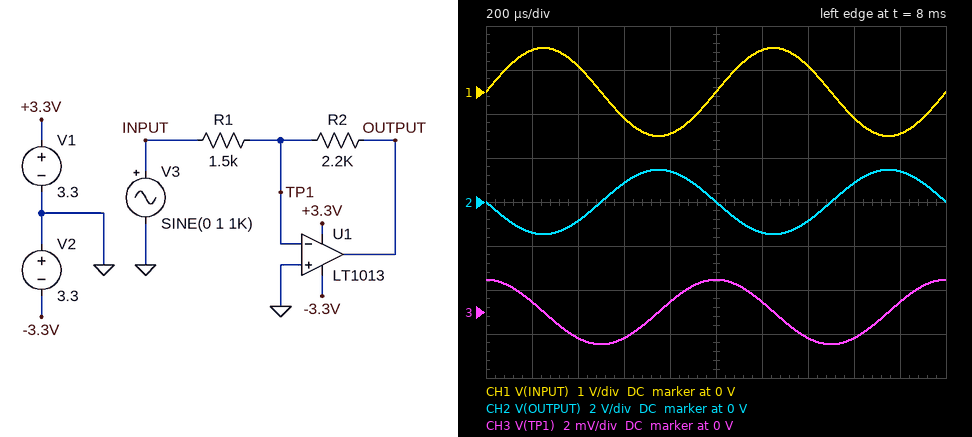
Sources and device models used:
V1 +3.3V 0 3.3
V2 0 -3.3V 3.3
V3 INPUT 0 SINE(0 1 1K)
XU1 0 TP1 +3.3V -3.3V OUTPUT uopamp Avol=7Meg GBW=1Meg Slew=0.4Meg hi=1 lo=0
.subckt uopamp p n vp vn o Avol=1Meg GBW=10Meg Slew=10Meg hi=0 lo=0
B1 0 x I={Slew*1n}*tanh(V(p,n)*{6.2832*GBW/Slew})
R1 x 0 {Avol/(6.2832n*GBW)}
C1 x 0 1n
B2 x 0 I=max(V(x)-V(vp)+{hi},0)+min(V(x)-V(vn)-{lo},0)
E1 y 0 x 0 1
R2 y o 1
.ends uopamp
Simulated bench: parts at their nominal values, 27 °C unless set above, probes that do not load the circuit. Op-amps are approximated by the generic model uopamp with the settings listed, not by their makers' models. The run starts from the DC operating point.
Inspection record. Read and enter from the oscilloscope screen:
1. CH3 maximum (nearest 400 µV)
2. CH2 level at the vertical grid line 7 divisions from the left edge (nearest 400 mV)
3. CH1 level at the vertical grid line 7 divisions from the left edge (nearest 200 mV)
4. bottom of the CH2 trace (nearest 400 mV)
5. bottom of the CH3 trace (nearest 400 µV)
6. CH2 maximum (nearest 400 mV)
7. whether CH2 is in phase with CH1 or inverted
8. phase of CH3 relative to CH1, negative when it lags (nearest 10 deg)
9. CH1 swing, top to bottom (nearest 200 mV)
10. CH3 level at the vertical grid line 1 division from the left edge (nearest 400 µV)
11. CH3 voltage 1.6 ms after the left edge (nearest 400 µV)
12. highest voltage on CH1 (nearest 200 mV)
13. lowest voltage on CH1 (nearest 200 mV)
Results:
1.6 mV
-800 mV
600 mV
-1.6 V
-1.6 mV
1.6 V
inverted
90 deg
2.0 V
400 µV
-1.2 mV
1.0 V
-1.0 V
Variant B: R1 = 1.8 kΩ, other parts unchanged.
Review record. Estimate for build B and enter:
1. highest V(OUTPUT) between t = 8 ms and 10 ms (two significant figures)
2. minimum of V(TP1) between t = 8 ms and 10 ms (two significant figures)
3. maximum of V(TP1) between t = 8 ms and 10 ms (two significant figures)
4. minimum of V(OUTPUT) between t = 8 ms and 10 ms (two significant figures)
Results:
1.2 V
-1.2 mV
1.2 mV
-1.2 V
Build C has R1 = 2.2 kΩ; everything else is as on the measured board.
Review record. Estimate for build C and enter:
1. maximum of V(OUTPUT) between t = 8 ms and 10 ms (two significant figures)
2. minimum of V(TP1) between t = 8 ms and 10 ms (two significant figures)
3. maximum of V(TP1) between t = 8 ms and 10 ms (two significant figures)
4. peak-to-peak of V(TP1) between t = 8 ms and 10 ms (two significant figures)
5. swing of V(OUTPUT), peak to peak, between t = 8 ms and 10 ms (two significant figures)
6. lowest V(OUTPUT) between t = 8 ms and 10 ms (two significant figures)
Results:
1.0 V
-1.0 mV
1.0 mV
2.0 mV
2.0 V
-1.0 V
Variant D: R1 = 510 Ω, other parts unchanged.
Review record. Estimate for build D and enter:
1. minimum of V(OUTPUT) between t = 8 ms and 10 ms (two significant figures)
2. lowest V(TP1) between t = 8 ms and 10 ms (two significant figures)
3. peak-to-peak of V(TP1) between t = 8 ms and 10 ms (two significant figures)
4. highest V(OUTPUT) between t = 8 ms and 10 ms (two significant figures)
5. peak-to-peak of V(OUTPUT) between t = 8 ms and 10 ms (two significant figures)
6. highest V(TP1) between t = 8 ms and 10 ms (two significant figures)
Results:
-3.3 V
-380 mV
570 mV
2.3 V
5.6 V
190 mV
